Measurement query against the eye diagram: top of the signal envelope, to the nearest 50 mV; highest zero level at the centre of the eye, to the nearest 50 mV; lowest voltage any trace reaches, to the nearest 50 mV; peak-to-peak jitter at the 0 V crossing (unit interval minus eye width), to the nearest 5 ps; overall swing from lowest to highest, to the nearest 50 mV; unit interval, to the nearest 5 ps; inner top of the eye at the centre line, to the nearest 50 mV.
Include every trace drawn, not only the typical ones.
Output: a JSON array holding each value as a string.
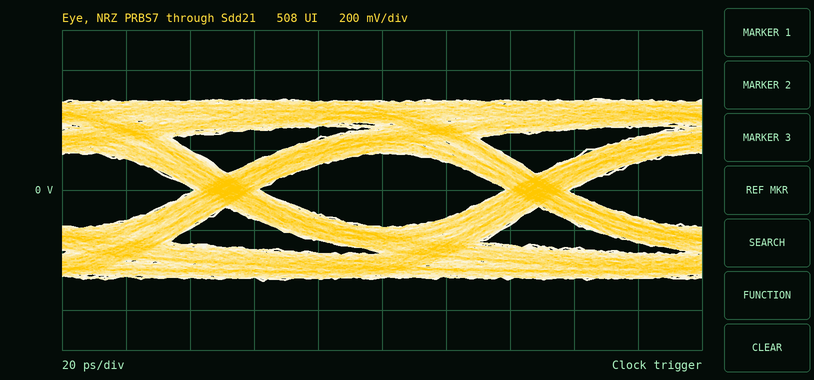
["450 mV", "-200 mV", "-450 mV", "20 ps", "900 mV", "95 ps", "200 mV"]
